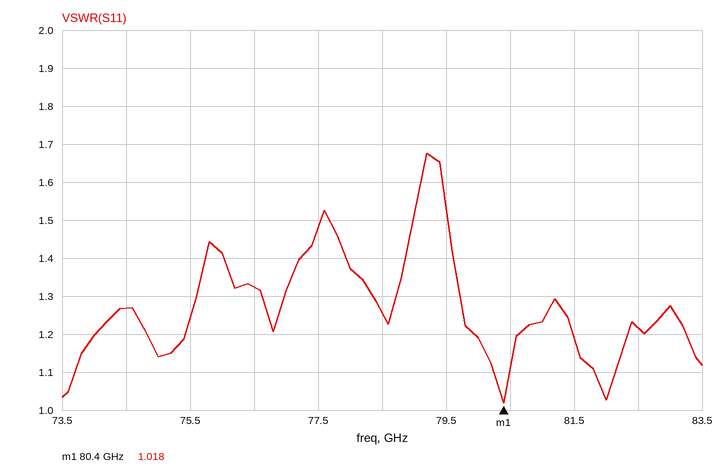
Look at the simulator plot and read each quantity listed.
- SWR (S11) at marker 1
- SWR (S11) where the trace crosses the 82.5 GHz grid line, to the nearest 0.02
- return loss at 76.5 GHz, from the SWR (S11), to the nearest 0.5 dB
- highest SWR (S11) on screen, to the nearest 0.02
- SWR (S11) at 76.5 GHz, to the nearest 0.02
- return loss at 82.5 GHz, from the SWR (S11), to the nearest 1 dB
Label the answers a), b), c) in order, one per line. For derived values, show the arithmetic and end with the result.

a) 1.018
b) 1.22
c) −20 log10((1.32 − 1)/(1.32 + 1)) ≈ 17.2 dB, so 17.0 dB to the nearest 0.5 dB
d) 1.68
e) 1.32
f) −20 log10((1.22 − 1)/(1.22 + 1)) ≈ 20 dB
